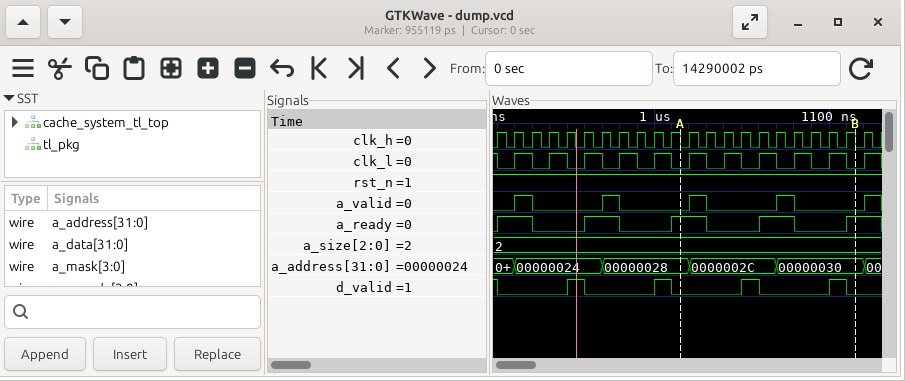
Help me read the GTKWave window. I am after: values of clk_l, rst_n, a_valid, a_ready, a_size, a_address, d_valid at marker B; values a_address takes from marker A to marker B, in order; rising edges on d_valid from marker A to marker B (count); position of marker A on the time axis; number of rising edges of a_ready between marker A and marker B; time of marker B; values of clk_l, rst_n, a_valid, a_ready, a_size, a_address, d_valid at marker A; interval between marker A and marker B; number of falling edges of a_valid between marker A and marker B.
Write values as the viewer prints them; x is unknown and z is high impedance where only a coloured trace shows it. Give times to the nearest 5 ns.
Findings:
clk_l=0, rst_n=1, a_valid=0, a_ready=1, a_size=2, a_address=00000030, d_valid=0
00000028, 0000002C, 00000030
2
1015 ns
2
1115 ns
clk_l=0, rst_n=1, a_valid=0, a_ready=1, a_size=2, a_address=00000028, d_valid=0
100 ns
2
